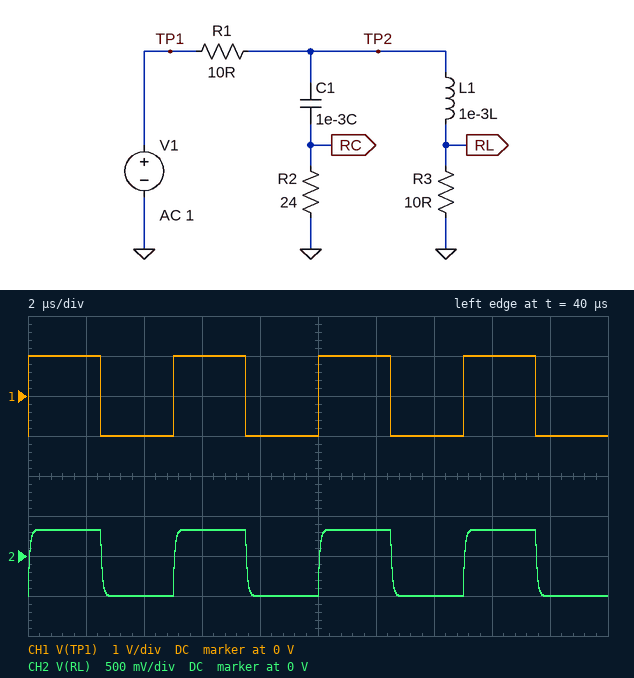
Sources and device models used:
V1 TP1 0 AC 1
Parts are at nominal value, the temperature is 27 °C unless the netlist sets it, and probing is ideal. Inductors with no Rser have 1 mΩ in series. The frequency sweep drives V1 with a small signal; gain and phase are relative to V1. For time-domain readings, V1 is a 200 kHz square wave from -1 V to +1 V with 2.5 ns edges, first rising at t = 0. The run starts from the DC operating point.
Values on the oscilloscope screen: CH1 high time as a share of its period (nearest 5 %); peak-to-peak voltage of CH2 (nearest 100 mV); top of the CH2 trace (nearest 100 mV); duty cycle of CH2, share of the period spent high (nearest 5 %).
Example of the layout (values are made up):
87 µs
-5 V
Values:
50 %
800 mV
300 mV
50 %
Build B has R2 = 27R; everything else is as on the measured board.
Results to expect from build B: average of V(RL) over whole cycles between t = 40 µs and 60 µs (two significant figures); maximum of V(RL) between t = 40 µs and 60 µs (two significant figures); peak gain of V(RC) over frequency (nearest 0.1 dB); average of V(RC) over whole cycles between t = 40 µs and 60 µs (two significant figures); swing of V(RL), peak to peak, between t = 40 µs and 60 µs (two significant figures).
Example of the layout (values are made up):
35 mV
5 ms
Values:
-78 mV
340 mV
-2.7 dB
420 mV
840 mV
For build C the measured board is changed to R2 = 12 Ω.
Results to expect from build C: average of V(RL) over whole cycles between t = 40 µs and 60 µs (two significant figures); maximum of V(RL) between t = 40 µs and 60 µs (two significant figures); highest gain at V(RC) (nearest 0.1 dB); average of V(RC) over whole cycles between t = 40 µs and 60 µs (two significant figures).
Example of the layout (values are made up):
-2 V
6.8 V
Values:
-150 mV
210 mV
-5.3 dB
350 mV
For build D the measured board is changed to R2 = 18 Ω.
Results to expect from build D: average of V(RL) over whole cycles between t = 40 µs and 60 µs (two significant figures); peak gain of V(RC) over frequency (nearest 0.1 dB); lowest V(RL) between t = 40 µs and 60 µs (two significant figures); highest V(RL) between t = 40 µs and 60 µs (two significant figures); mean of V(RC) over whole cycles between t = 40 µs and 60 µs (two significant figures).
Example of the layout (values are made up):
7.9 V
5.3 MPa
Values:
-110 mV
-3.8 dB
-500 mV
280 mV
390 mV
